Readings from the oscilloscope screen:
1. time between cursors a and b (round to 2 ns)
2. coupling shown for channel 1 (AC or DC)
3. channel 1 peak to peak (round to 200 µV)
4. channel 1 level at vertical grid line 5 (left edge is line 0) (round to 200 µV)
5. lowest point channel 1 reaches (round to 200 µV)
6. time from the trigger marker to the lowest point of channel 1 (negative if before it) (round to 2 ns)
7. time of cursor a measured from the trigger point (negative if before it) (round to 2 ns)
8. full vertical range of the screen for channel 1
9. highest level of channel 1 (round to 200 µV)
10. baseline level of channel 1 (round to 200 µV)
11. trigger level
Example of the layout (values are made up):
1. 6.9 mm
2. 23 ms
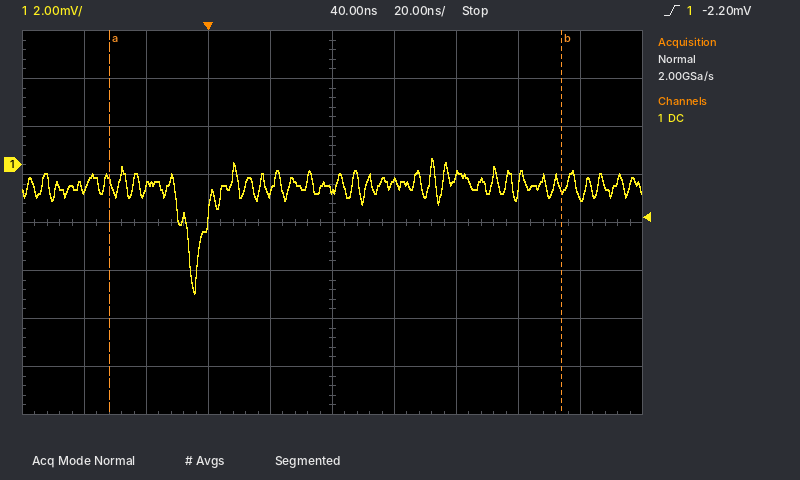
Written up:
1. 146 ns
2. DC
3. 5.6 mV
4. -1.0 mV
5. -5.4 mV
6. -4 ns
7. -32 ns
8. 16 mV
9. 200 µV
10. -800 µV
11. -2.20 mV
